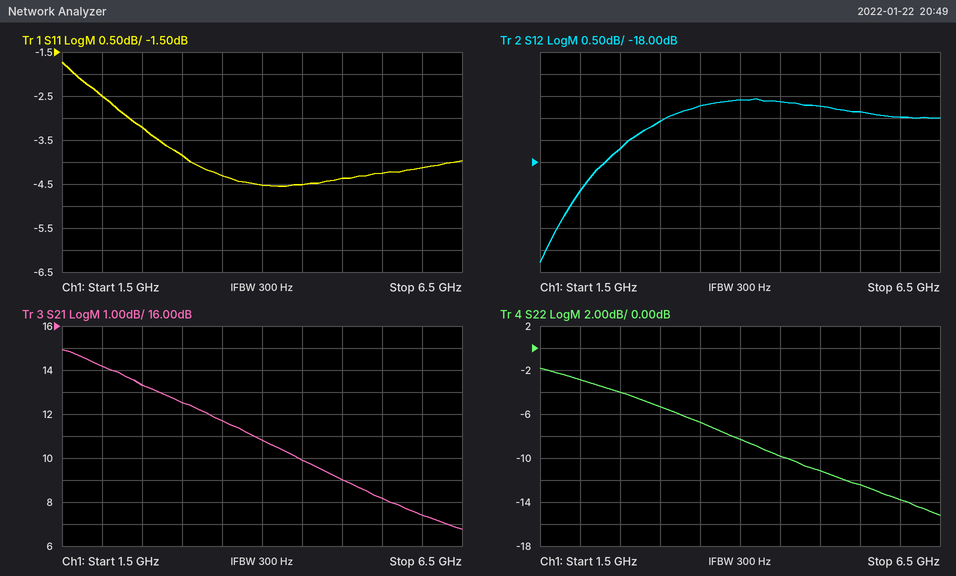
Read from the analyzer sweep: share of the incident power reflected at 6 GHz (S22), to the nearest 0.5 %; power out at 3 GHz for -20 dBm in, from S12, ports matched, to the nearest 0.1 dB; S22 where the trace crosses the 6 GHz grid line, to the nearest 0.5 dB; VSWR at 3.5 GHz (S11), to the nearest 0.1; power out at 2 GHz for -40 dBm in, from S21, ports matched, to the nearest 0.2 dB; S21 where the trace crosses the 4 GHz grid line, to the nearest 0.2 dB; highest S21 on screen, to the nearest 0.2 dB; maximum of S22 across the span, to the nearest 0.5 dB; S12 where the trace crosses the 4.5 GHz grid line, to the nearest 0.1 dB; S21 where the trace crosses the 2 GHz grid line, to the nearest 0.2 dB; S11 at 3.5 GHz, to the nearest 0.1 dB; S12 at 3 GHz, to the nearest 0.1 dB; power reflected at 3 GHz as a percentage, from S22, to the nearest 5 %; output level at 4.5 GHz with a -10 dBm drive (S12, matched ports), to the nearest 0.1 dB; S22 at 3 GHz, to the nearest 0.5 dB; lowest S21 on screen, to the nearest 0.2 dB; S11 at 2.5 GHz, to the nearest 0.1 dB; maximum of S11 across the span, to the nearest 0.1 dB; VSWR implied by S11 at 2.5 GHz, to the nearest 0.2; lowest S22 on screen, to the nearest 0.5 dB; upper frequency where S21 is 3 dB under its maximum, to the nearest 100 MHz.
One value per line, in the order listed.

4.0 %
-37.1 dBm
-14.0 dB
4.1
-25.8 dBm
10.8 dB
15.0 dB
-2.0 dB
-16.6 dB
14.2 dB
-4.3 dB
-17.1 dB
30 %
-26.6 dBm
-5.5 dB
6.8 dB
-3.2 dB
-1.7 dB
5.4
-15.0 dB
3.4 GHz
